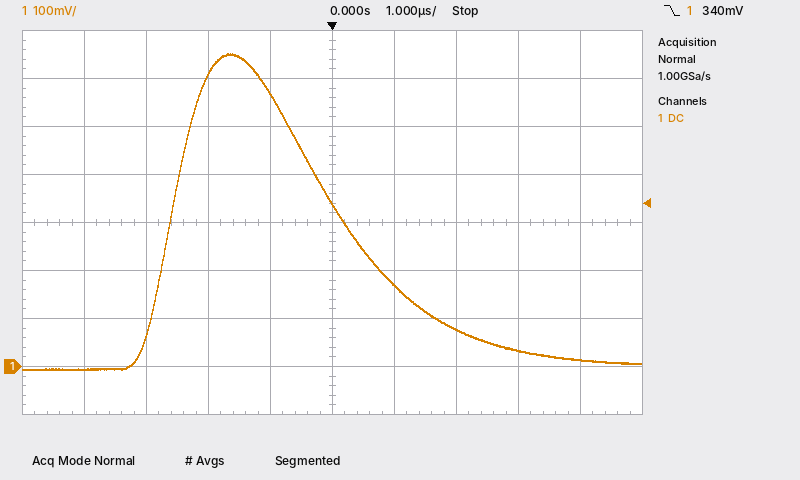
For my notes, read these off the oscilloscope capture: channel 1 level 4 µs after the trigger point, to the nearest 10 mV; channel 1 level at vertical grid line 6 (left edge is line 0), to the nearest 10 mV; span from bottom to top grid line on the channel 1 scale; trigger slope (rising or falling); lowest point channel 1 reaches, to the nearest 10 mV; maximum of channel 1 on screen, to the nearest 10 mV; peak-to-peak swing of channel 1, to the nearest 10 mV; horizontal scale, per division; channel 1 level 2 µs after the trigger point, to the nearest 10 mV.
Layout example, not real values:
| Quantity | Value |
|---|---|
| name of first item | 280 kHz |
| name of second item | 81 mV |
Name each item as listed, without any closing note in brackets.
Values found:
| Quantity | Value |
|---|---|
| channel 1 level 4 µs after the trigger point, to the nearest 10 mV | 10 mV |
| channel 1 level at vertical grid line 6 (left edge is line 0), to the nearest 10 mV | 170 mV |
| span from bottom to top grid line on the channel 1 scale | 800 mV |
| trigger slope | falling |
| lowest point channel 1 reaches, to the nearest 10 mV | -10 mV |
| maximum of channel 1 on screen, to the nearest 10 mV | 650 mV |
| peak-to-peak swing of channel 1, to the nearest 10 mV | 660 mV |
| horizontal scale, per division | 1 µs |
| channel 1 level 2 µs after the trigger point, to the nearest 10 mV | 80 mV |
